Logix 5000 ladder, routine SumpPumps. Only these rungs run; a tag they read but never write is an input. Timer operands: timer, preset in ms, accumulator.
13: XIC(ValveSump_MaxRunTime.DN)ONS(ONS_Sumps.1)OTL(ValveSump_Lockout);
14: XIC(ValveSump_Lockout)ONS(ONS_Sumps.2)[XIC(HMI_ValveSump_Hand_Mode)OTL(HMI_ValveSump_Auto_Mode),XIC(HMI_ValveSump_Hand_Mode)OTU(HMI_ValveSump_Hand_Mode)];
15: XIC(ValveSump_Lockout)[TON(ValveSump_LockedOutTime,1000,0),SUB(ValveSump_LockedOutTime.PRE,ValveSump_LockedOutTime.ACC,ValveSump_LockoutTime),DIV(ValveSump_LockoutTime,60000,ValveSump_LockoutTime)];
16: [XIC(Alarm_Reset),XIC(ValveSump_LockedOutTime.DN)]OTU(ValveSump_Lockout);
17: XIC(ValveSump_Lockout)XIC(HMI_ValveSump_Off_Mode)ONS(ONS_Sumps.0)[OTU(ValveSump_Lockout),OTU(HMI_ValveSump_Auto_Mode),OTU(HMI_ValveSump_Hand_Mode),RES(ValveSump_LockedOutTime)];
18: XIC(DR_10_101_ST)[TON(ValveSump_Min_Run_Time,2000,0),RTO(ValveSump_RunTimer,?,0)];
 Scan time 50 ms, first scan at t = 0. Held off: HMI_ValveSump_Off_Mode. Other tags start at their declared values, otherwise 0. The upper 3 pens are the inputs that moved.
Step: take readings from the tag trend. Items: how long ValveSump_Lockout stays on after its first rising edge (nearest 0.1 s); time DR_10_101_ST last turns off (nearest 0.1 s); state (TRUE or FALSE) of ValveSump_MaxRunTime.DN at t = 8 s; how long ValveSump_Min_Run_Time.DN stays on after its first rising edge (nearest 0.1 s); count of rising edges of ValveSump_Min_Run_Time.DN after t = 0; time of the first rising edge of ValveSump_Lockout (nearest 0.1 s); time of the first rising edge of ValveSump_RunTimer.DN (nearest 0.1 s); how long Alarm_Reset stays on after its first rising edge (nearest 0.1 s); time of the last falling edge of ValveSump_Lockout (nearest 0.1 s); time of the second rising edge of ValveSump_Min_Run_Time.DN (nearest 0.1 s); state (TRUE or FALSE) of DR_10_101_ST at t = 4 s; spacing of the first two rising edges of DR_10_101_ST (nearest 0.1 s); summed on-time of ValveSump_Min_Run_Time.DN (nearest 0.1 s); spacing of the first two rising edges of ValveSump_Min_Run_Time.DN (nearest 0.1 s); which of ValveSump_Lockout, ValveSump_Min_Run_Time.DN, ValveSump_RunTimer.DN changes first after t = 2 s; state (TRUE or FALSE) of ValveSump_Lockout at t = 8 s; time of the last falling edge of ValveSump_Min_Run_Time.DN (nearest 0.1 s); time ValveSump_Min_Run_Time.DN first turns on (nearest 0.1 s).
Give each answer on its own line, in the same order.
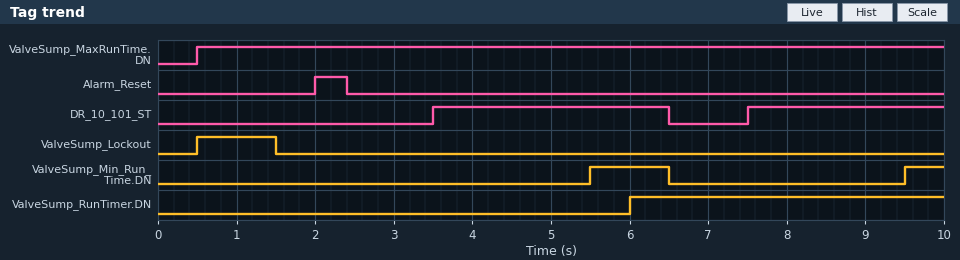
1.0 s
6.5 s
TRUE
1.0 s
2
0.5 s
6.0 s
0.4 s
1.5 s
9.5 s
TRUE
4.0 s
1.5 s
4.0 s
ValveSump_Min_Run_Time.DN
FALSE
6.5 s
5.5 s
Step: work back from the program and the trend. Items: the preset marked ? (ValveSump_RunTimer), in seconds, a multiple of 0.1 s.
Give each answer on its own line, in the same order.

2.5 s
